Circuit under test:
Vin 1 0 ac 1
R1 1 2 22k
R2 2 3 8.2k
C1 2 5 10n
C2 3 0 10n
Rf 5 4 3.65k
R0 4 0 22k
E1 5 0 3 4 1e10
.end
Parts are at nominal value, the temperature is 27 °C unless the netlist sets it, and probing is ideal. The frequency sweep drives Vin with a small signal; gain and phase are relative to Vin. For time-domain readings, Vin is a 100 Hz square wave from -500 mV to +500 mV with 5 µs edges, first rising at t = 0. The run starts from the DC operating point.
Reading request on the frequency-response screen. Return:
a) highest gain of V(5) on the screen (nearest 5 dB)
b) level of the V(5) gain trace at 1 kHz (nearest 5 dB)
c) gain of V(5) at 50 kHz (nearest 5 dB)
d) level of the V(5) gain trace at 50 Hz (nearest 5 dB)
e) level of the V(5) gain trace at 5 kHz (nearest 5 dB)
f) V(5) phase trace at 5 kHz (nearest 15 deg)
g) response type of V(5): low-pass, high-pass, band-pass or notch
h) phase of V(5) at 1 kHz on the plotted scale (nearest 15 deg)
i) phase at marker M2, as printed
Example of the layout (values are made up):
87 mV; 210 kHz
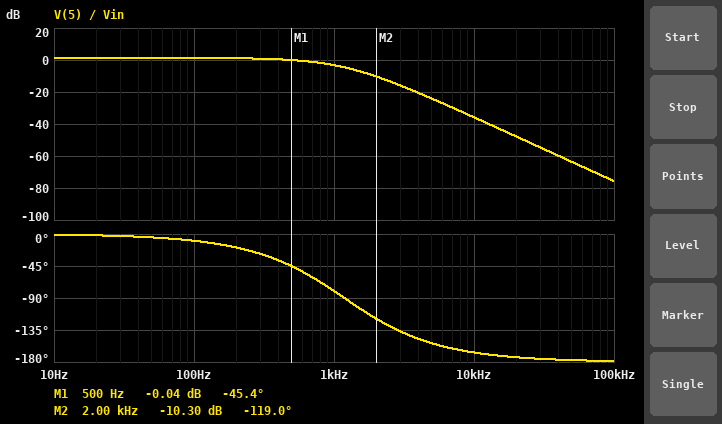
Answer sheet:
0 dB; -5 dB; -65 dB; 0 dB; -25 dB; -150 deg; low-pass; -75 deg; -119.0 deg
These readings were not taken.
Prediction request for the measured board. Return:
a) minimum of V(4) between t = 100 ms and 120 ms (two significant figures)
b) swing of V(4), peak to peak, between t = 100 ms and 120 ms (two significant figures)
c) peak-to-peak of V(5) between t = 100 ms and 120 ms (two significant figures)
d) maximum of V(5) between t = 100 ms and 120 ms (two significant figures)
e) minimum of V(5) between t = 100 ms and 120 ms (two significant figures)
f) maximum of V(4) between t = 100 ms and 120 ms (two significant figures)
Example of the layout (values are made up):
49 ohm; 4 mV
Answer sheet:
-500 mV; 1.0 V; 1.2 V; 580 mV; -580 mV; 500 mV
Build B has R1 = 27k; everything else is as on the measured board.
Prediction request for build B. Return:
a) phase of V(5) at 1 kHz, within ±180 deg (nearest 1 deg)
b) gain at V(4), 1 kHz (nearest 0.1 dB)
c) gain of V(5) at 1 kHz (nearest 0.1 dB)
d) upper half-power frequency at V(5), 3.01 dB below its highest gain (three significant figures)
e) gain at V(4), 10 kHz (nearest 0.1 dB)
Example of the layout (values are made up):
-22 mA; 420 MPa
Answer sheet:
-86 deg; -5.7 dB; -4.4 dB; 658 Hz; -38.9 dB
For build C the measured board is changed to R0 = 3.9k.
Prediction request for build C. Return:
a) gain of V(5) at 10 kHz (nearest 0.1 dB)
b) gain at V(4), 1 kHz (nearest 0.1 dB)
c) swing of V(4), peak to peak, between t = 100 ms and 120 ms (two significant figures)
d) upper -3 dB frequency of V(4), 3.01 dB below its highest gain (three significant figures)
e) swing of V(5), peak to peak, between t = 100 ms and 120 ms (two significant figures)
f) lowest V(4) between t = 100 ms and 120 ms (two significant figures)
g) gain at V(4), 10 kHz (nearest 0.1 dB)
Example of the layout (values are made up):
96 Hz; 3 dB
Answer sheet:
-31.2 dB; 3.5 dB; 1.6 V; 1.41 kHz; 3.1 V; -800 mV; -37.0 dB
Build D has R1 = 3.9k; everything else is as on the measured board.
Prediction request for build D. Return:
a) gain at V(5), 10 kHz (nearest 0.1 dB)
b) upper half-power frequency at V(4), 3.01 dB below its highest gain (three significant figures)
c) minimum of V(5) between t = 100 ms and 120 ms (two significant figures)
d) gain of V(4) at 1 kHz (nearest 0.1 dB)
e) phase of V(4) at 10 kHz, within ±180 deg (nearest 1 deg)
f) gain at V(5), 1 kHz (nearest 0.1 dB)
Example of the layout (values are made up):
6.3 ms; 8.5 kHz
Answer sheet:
-21.4 dB; 1.78 kHz; -580 mV; -1.1 dB; -148 deg; 0.3 dB
